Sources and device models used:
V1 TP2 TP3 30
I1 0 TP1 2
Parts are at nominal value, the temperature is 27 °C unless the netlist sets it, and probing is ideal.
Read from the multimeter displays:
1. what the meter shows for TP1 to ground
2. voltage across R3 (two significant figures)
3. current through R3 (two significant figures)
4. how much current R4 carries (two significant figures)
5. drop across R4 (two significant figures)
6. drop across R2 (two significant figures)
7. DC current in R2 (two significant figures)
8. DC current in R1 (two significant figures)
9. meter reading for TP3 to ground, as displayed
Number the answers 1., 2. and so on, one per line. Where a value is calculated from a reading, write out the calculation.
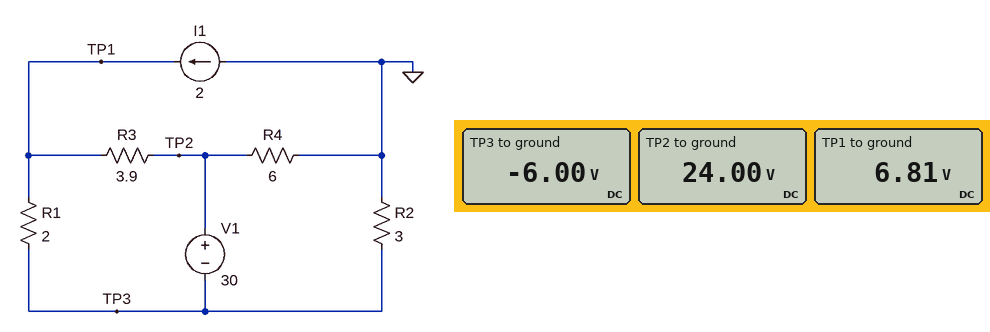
1. 6.81 V
2. 24 V - 6.81 V = 17 V
3. (24 V - 6.81 V) / 3.9 Ω = 4.4 A
4. (24 V) / 6 Ω = 4.0 A
5. 24 V = 24 V
6. 0 V - (-6 V) = 6.0 V
7. (0 V - (-6 V)) / 3 Ω = 2.0 A
8. (6.81 V - (-6 V)) / 2 Ω = 6.4 A
9. -6.00 V
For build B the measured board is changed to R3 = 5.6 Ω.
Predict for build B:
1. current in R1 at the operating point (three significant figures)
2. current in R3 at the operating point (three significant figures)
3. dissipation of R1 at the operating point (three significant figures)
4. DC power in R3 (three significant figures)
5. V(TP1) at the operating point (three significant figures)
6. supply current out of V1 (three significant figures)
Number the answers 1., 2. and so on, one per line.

1. 5.42 A
2. 3.42 A
3. 58.8 W
4. 65.5 W
5. 4.84 V
6. 7.42 A
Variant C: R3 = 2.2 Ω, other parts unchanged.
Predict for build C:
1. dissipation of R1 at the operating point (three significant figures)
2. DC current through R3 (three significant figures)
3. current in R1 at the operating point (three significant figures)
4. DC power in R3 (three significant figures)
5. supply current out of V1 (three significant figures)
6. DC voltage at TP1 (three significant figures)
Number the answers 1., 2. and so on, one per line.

1. 134 W
2. 6.19 A
3. 8.19 A
4. 84.3 W
5. 10.2 A
6. 10.4 V
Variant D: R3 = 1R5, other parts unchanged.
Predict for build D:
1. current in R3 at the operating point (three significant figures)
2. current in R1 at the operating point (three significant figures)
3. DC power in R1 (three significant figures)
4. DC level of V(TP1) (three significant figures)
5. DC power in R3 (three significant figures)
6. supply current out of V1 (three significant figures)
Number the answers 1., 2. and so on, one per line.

1. 7.43 A
2. 9.43 A
3. 178 W
4. 12.9 V
5. 82.8 W
6. 11.4 A
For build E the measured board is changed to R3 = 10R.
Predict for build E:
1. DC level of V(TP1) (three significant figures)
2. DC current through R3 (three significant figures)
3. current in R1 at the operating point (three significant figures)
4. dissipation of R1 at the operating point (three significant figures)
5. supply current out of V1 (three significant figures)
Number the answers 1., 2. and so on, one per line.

1. 2.33 V
2. 2.17 A
3. 4.17 A
4. 34.7 W
5. 6.17 A
